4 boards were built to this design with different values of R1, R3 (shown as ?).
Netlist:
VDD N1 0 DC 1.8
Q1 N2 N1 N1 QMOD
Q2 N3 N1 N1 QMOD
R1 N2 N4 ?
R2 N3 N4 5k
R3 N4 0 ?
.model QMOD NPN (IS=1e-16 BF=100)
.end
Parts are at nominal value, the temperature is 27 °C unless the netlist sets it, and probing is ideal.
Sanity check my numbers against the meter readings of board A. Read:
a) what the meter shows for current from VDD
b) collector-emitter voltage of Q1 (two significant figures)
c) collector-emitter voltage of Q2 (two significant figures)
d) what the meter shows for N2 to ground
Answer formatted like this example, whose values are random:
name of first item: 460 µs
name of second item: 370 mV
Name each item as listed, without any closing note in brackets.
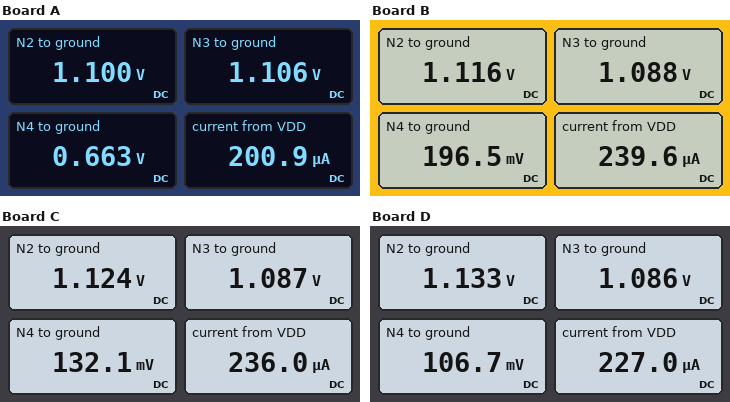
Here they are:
what the meter shows for current from VDD: 200.9 µA
collector-emitter voltage of Q1: -700 mV
collector-emitter voltage of Q2: -690 mV
what the meter shows for N2 to ground: 1.100 V
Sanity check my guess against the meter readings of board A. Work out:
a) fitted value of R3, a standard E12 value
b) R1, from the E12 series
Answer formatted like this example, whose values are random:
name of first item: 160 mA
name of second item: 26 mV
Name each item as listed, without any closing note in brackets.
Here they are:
fitted value of R3, a standard E12 value: 3.3 kΩ
R1, from the E12 series: 3.9 kΩ
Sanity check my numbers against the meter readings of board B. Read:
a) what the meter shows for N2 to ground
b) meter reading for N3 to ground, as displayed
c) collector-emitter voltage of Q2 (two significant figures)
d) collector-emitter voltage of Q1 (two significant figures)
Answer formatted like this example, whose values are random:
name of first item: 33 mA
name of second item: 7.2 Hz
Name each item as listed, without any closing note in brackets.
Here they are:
what the meter shows for N2 to ground: 1.116 V
meter reading for N3 to ground, as displayed: 1.088 V
collector-emitter voltage of Q2: -710 mV
collector-emitter voltage of Q1: -680 mV
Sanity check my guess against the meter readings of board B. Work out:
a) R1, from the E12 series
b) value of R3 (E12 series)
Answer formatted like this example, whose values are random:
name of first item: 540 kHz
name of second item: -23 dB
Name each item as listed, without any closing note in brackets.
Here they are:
R1, from the E12 series: 15 kΩ
value of R3: 820 Ω
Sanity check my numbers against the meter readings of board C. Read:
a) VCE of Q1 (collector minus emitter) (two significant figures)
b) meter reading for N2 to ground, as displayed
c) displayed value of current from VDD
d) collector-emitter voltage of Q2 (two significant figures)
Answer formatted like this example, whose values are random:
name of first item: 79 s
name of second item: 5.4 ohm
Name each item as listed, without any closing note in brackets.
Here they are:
VCE of Q1 (collector minus emitter): -680 mV
meter reading for N2 to ground, as displayed: 1.124 V
displayed value of current from VDD: 236.0 µA
collector-emitter voltage of Q2: -710 mV
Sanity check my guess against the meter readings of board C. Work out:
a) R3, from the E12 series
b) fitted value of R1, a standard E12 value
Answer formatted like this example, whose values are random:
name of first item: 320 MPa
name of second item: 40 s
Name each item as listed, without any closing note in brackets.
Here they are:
R3, from the E12 series: 560 Ω
fitted value of R1, a standard E12 value: 22 kΩ
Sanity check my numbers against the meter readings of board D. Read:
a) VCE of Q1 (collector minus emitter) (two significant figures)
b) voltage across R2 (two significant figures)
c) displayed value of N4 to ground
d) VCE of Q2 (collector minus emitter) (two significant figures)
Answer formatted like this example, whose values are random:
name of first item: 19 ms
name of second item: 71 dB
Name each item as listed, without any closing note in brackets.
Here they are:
VCE of Q1 (collector minus emitter): -670 mV
voltage across R2: 980 mV
displayed value of N4 to ground: 106.7 mV
VCE of Q2 (collector minus emitter): -710 mV
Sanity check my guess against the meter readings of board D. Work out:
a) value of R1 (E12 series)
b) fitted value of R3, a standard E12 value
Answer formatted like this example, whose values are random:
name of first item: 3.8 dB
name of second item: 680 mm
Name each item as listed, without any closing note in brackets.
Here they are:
value of R1: 33 kΩ
fitted value of R3, a standard E12 value: 470 Ω
